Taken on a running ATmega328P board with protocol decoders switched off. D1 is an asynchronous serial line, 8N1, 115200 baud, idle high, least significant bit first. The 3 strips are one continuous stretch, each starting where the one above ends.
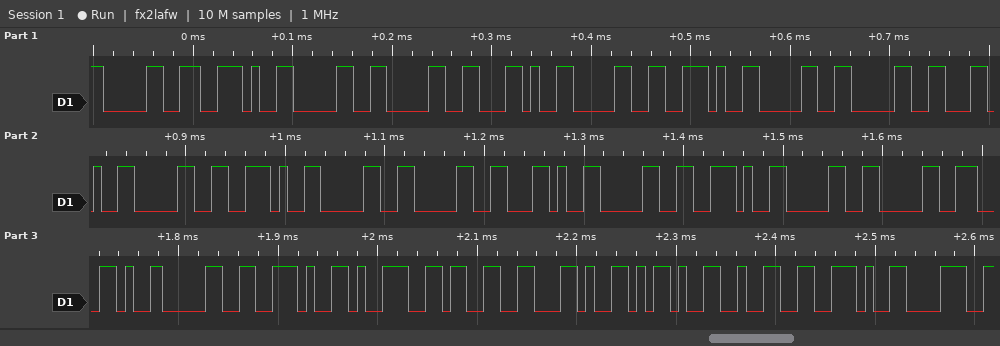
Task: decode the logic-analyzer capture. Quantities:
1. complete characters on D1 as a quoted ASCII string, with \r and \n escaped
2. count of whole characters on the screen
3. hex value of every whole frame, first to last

"0.00,0.00,0.00,0.00,0.93,-2.8"
29
30 2E 30 30 2C 30 2E 30 30 2C 30 2E 30 30 2C 30 2E 30 30 2C 30 2E 39 33 2C 2D 32 2E 38
